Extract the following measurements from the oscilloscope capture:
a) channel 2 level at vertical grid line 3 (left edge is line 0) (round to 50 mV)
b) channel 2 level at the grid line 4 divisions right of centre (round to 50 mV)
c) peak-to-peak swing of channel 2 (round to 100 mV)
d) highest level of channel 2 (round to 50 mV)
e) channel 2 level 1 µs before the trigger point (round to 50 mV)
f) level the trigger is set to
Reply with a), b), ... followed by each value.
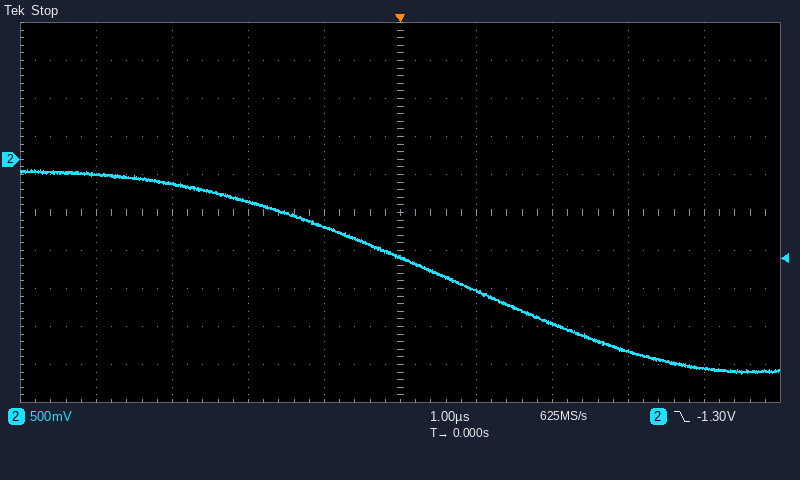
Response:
a) -550 mV
b) -2.75 V
c) 2.70 V
d) -150 mV
e) -900 mV
f) -1.30 V
